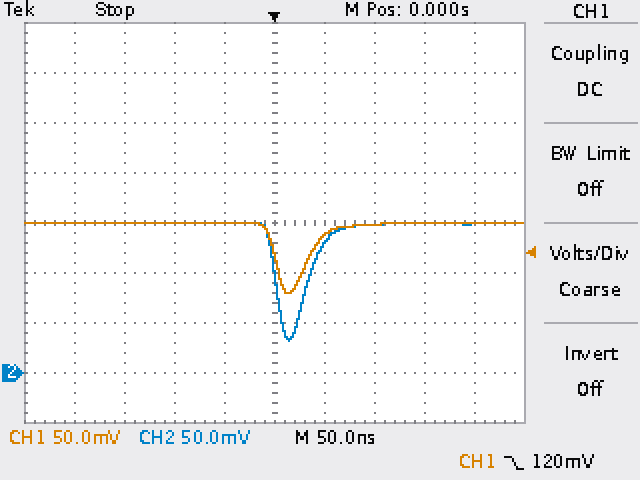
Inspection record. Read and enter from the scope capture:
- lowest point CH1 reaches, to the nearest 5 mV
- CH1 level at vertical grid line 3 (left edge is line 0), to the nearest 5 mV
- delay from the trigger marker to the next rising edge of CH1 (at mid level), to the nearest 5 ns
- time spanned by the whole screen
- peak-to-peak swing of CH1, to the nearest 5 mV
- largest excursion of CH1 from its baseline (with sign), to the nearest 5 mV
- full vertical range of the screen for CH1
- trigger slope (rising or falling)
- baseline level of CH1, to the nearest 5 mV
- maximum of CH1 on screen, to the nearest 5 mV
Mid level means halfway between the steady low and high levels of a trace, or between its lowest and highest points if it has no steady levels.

80 mV
150 mV
35 ns
500 ns
70 mV
-70 mV
400 mV
falling
150 mV
150 mV
